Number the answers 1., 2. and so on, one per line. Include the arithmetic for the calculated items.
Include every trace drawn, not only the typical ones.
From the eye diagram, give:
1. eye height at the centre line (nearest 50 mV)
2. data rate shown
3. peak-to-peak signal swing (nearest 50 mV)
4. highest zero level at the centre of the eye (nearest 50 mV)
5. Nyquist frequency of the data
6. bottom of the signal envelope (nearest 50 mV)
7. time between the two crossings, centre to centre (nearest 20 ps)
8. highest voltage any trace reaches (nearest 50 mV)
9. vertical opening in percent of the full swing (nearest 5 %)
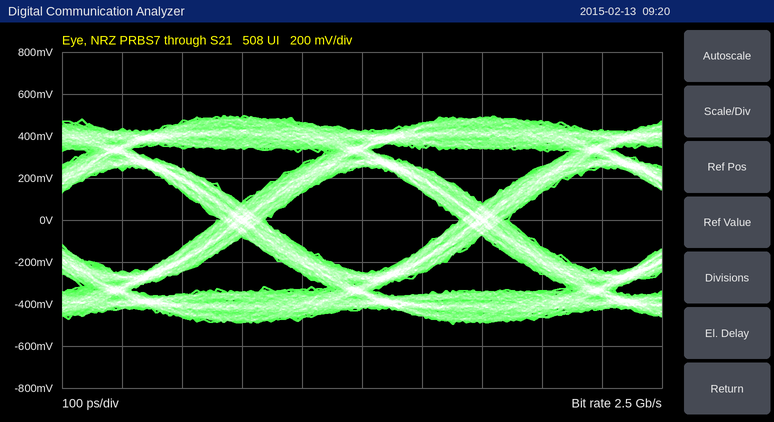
1. 500 mV
2. 2.5 Gb/s
3. 1.00 V
4. -250 mV
5. 1.25 GHz
6. -500 mV
7. 400 ps
8. 500 mV
9. 500 mV / 1.00 V ≈ 50 %
